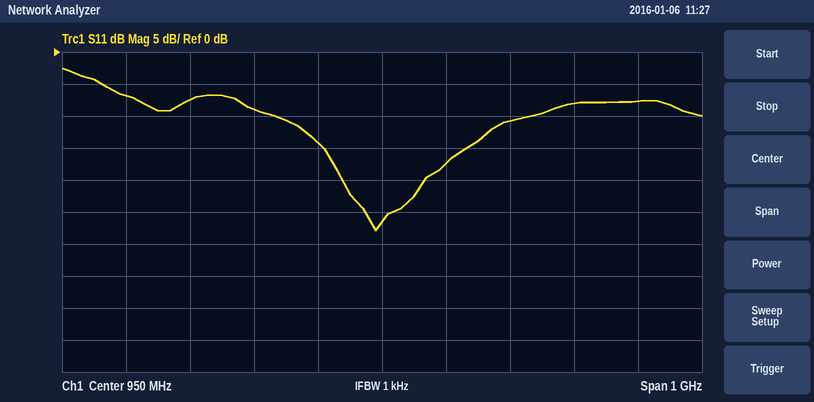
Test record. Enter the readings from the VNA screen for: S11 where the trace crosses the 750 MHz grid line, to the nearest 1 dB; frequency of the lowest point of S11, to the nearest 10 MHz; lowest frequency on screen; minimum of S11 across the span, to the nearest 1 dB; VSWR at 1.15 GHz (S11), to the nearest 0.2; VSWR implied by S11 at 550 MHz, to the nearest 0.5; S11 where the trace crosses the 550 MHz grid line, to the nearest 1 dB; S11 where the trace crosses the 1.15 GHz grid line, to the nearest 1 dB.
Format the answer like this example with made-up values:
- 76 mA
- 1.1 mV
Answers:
- -9 dB
- 940 MHz
- 450 MHz
- -28 dB
- 1.8
- 2.5
- -7 dB
- -11 dB
